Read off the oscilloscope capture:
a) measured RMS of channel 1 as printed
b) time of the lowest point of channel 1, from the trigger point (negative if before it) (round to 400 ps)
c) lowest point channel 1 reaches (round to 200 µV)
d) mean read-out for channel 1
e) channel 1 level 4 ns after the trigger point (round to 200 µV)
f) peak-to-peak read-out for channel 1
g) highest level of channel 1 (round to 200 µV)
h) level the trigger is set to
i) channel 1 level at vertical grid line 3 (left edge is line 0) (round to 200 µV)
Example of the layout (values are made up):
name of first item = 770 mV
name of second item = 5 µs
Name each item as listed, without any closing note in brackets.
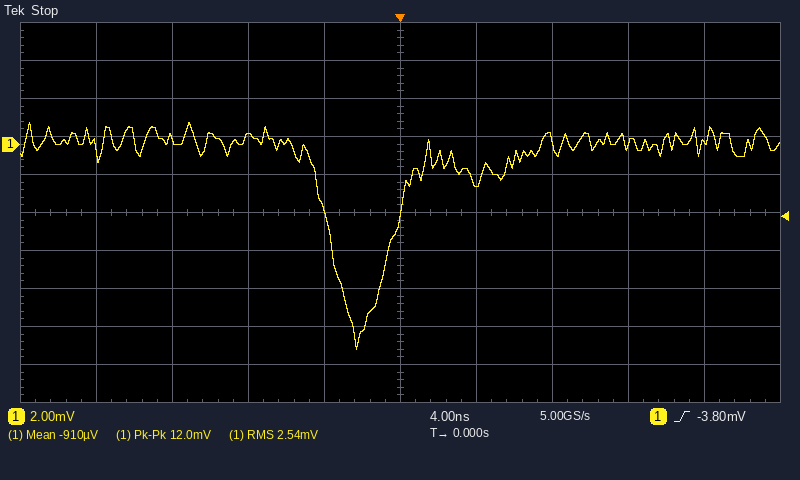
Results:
measured RMS of channel 1 as printed = 2.54 mV
time of the lowest point of channel 1, from the trigger point (negative if before it) = -2.4 ns
lowest point channel 1 reaches = -10.8 mV
mean read-out for channel 1 = -910 µV
channel 1 level 4 ns after the trigger point = -2.0 mV
peak-to-peak read-out for channel 1 = 12.0 mV
highest level of channel 1 = 1.2 mV
level the trigger is set to = -3.80 mV
channel 1 level at vertical grid line 3 (left edge is line 0) = 400 µV
